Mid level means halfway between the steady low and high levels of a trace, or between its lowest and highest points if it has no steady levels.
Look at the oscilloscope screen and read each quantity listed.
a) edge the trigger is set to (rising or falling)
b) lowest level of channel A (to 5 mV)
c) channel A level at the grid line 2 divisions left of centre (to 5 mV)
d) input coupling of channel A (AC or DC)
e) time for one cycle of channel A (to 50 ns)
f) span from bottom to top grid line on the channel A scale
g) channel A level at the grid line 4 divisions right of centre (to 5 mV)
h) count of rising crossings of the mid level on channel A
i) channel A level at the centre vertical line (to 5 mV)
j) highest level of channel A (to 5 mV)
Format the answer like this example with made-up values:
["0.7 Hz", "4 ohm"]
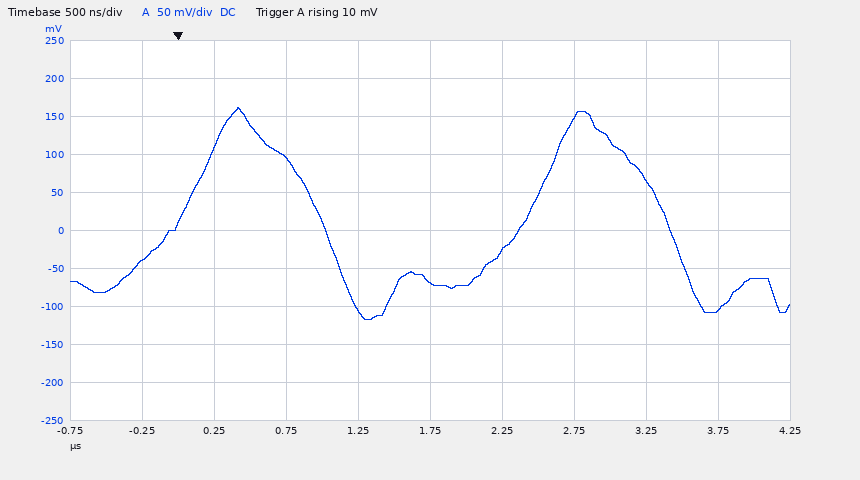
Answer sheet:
["rising", "-115 mV", "95 mV", "DC", "2.40 µs", "500 mV", "-105 mV", "2", "-70 mV", "160 mV"]
